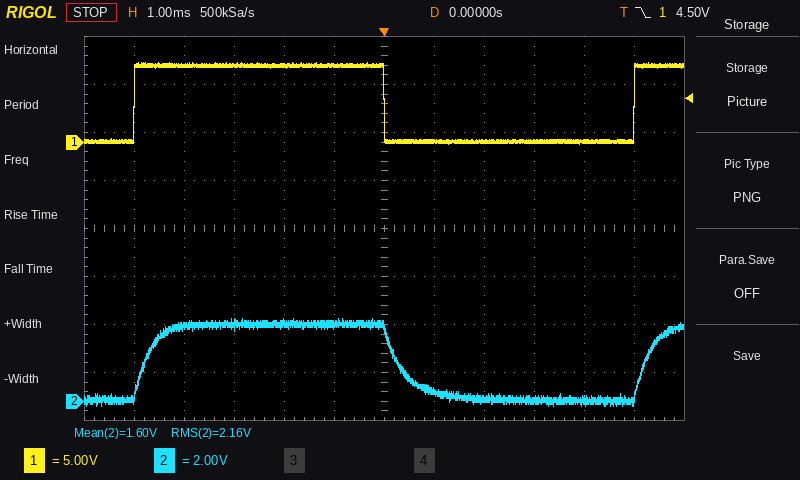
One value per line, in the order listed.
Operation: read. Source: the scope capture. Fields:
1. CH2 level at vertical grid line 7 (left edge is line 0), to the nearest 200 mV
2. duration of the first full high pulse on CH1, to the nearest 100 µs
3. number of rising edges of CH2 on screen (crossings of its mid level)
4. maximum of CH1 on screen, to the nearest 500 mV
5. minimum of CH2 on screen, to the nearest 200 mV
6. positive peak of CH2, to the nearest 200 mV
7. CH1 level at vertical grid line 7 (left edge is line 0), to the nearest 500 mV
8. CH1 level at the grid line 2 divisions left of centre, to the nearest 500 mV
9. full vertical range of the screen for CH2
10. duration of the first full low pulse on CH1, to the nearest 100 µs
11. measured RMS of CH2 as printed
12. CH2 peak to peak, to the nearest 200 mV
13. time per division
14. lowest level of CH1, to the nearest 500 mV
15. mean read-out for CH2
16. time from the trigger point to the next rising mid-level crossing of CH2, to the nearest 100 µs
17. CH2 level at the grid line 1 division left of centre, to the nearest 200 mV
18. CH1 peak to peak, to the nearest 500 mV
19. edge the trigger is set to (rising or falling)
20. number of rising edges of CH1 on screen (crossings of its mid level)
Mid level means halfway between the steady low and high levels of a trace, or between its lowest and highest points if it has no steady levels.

400 mV
5.0 ms
2
8.5 V
-200 mV
3.4 V
0.0 V
8.0 V
16 V
5.0 ms
2.16 V
3.6 V
1 ms
0.0 V
1.60 V
5.2 ms
3.2 V
8.5 V
falling
2
